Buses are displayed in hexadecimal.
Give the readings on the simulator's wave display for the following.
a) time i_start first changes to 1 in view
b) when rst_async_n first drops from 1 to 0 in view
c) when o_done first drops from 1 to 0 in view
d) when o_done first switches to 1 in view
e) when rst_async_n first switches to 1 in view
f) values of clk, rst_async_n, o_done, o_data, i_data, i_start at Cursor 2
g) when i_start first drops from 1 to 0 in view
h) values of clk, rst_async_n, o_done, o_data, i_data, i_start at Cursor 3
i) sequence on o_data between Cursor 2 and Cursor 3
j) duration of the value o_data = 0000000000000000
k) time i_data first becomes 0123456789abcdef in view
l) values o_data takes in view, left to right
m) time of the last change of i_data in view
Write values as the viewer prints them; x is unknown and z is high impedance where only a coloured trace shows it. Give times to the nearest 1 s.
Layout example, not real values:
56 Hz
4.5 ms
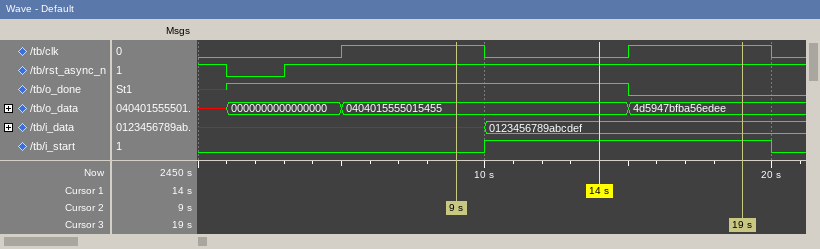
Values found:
10 s
1 s
15 s
1 s
3 s
clk=1, rst_async_n=1, o_done=1, o_data=0404015555015455, i_data=x, i_start=0
20 s
clk=1, rst_async_n=1, o_done=0, o_data=4d5947bfba56edee, i_data=0123456789abcdef, i_start=1
0404015555015455, 4d5947bfba56edee
4 s
10 s
x, 0000000000000000, 0404015555015455, 4d5947bfba56edee
10 s
